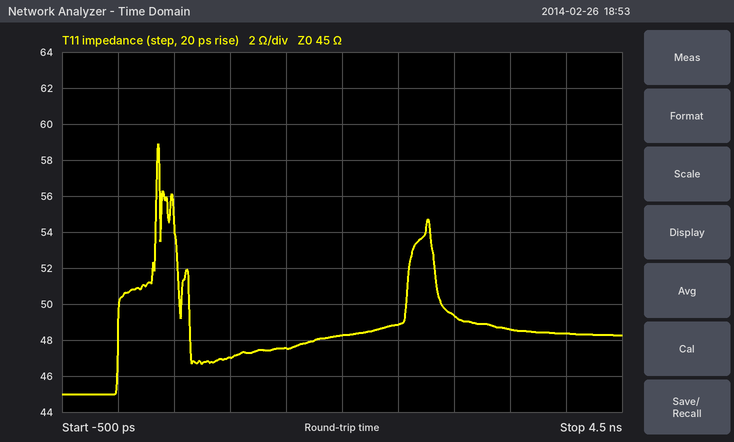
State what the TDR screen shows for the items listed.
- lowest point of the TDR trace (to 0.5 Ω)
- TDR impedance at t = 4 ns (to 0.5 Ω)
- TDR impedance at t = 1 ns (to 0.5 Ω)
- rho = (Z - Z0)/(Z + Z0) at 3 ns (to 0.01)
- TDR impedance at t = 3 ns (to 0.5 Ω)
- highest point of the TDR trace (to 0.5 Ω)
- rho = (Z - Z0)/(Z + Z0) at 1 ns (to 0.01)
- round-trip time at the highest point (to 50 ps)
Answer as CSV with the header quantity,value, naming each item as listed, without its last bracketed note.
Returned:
quantity,value
lowest point of the TDR trace,45.0 Ω
TDR impedance at t = 4 ns,48.5 Ω
TDR impedance at t = 1 ns,47.0 Ω
rho = (Z - Z0)/(Z + Z0) at 3 ns,+0.05
TDR impedance at t = 3 ns,49.5 Ω
highest point of the TDR trace,59.0 Ω
rho = (Z - Z0)/(Z + Z0) at 1 ns,+0.02
round-trip time at the highest point,350 ps
